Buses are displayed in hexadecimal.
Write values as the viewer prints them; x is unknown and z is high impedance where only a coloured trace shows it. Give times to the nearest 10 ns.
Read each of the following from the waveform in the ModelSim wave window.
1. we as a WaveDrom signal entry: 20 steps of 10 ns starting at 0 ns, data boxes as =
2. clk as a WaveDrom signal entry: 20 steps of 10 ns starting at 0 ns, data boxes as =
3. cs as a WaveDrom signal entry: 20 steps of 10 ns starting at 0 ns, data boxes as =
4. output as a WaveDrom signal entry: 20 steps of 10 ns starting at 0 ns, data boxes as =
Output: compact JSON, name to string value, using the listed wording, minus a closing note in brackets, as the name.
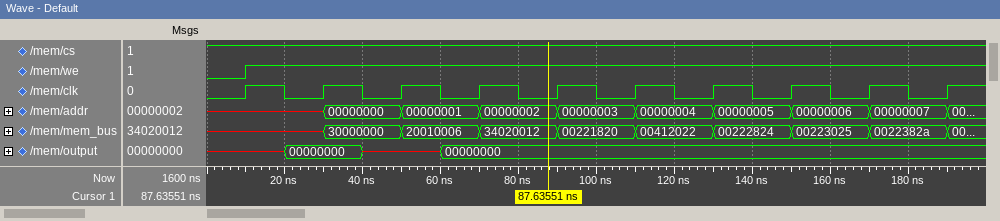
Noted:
{"we as a WaveDrom signal entry: 20 steps of 10 ns starting at 0 ns, data boxes as =": "{name: 'we', wave: '01..................'}", "clk as a WaveDrom signal entry: 20 steps of 10 ns starting at 0 ns, data boxes as =": "{name: 'clk', wave: '01010101010101010101'}", "cs as a WaveDrom signal entry: 20 steps of 10 ns starting at 0 ns, data boxes as =": "{name: 'cs', wave: '1...................'}", "output as a WaveDrom signal entry: 20 steps of 10 ns starting at 0 ns, data boxes as =": "{name: 'output', wave: 'x.=.x.=.............', data: '00000000 00000000'}"}
